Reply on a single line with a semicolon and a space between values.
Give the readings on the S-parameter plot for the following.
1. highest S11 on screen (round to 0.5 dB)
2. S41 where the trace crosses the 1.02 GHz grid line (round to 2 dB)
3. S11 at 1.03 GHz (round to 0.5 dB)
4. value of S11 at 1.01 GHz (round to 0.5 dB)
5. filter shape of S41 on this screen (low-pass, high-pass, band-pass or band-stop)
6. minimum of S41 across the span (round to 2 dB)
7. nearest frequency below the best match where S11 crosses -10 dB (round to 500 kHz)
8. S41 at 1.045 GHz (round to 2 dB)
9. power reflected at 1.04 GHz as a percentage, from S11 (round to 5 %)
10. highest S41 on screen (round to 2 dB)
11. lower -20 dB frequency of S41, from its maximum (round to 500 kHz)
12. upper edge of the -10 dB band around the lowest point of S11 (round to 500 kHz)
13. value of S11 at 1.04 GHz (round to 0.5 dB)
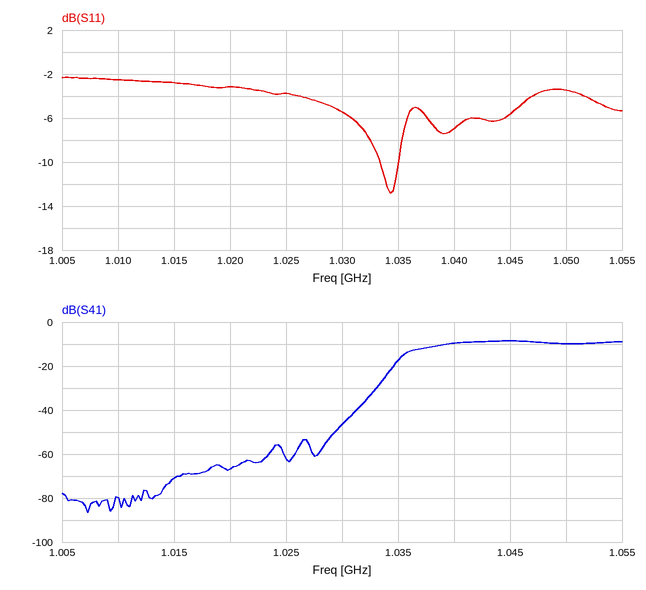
-2.5 dB; -66 dB; -5.5 dB; -2.5 dB; high-pass; -86 dB; 1.0335 GHz; -8 dB; 20 %; -8 dB; 1.0335 GHz; 1.0350 GHz; -7.0 dB
